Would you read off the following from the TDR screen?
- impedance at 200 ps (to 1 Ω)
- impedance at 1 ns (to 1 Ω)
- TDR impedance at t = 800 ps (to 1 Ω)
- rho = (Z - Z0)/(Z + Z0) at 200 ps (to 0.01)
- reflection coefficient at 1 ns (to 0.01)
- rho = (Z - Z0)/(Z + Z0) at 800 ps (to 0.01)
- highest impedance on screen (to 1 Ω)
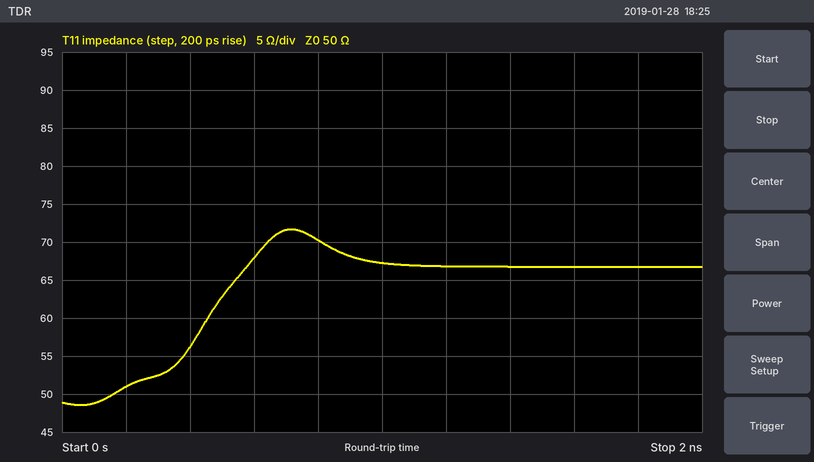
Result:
51 Ω
67 Ω
70 Ω
+0.01
+0.15
+0.17
72 Ω
